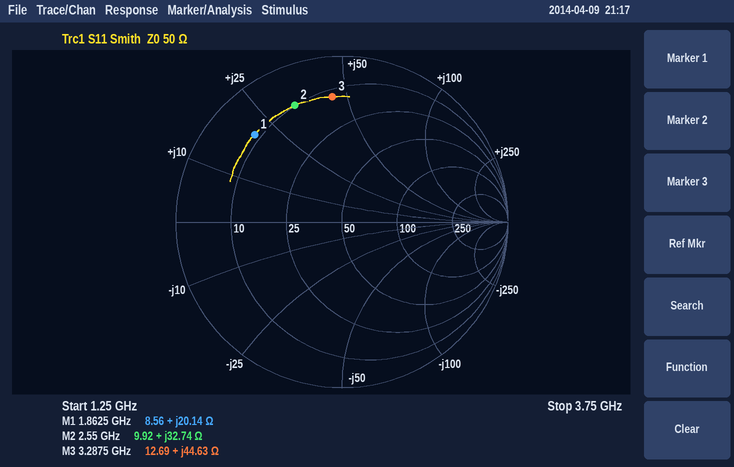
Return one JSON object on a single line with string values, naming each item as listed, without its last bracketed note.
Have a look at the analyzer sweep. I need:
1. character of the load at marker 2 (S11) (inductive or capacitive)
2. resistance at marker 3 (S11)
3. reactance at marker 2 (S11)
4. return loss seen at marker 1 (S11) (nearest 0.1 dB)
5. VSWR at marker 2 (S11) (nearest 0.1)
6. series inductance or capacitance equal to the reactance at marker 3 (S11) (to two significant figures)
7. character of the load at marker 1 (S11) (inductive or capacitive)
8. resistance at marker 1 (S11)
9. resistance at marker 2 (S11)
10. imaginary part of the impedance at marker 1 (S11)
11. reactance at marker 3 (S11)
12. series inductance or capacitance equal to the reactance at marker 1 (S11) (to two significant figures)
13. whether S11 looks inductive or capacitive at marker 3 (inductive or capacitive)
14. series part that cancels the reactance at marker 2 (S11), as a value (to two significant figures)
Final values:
{"character of the load at marker 2 (S11)": "inductive", "resistance at marker 3": "12.69 Ω", "reactance at marker 2": "+32.74 Ω", "return loss seen at marker 1 (S11)": "2.6 dB", "VSWR at marker 2 (S11)": "7.3", "series inductance or capacitance equal to the reactance at marker 3 (S11)": "2.2 nH", "character of the load at marker 1 (S11)": "inductive", "resistance at marker 1": "8.56 Ω", "resistance at marker 2": "9.92 Ω", "imaginary part of the impedance at marker 1": "+20.14 Ω", "reactance at marker 3": "+44.63 Ω", "series inductance or capacitance equal to the reactance at marker 1 (S11)": "1.7 nH", "whether S11 looks inductive or capacitive at marker 3": "inductive", "series part that cancels the reactance at marker 2 (S11), as a value": "1.9 pF"}
